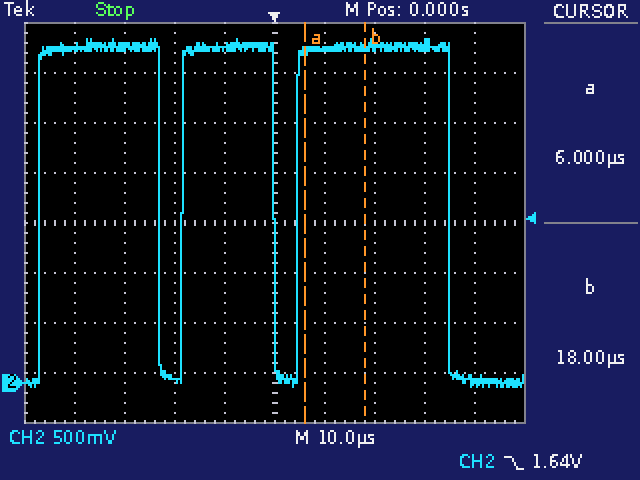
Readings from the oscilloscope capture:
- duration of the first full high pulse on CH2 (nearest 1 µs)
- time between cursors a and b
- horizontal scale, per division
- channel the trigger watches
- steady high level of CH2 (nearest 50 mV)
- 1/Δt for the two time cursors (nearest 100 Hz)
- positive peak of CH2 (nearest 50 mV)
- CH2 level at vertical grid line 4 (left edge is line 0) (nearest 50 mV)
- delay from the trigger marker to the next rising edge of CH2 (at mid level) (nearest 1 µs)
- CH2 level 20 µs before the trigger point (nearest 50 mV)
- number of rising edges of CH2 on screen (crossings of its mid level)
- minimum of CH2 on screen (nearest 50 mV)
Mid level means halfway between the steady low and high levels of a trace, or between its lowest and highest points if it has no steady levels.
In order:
24 µs
12 µs
10 µs
CH2
3.35 V
83.3 kHz
3.45 V
3.35 V
5 µs
50 mV
3
-50 mV
